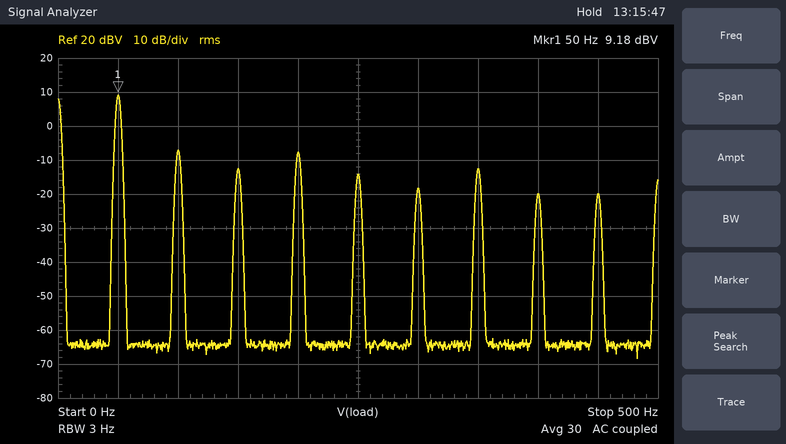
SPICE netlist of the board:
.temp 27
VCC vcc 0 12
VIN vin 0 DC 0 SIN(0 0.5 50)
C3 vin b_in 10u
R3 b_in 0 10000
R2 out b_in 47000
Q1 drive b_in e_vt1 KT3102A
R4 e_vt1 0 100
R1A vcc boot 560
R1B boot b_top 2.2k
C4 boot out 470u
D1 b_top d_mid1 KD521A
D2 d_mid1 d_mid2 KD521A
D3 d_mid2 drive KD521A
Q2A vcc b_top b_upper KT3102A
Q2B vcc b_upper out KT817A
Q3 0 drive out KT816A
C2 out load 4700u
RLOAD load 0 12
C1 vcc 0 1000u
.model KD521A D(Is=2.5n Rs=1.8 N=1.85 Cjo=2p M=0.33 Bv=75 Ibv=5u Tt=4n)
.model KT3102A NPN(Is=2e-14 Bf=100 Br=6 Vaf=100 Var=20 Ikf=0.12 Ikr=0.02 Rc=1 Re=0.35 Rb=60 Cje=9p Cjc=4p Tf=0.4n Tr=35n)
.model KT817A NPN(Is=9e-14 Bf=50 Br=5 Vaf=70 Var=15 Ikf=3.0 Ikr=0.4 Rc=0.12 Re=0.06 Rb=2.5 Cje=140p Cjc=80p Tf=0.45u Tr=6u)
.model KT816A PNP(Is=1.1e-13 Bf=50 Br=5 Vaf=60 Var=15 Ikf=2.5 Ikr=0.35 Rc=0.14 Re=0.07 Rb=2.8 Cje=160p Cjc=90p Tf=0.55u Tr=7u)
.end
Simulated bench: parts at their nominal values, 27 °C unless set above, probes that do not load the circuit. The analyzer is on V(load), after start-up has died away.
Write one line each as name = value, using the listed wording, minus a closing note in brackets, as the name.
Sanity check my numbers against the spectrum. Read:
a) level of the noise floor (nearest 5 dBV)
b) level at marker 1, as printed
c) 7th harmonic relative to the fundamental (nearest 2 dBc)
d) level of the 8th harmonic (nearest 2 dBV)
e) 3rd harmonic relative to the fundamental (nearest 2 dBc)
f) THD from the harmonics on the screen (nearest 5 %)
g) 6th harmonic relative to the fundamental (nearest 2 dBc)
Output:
level of the noise floor = -65 dBV
level at marker 1, as printed = 9.18 dBV
7th harmonic relative to the fundamental = -22 dBc
level of the 8th harmonic = -20 dBV
3rd harmonic relative to the fundamental = -22 dBc
THD from the harmonics on the screen = 25 %
6th harmonic relative to the fundamental = -28 dBc
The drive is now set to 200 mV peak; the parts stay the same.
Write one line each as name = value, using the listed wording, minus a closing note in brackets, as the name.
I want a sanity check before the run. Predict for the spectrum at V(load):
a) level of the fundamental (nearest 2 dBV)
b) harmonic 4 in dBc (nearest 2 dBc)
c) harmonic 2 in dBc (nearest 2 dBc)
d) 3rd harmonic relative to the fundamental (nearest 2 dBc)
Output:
level of the fundamental = 4 dBV
harmonic 4 in dBc = -14 dBc
harmonic 2 in dBc = -6 dBc
3rd harmonic relative to the fundamental = -10 dBc
